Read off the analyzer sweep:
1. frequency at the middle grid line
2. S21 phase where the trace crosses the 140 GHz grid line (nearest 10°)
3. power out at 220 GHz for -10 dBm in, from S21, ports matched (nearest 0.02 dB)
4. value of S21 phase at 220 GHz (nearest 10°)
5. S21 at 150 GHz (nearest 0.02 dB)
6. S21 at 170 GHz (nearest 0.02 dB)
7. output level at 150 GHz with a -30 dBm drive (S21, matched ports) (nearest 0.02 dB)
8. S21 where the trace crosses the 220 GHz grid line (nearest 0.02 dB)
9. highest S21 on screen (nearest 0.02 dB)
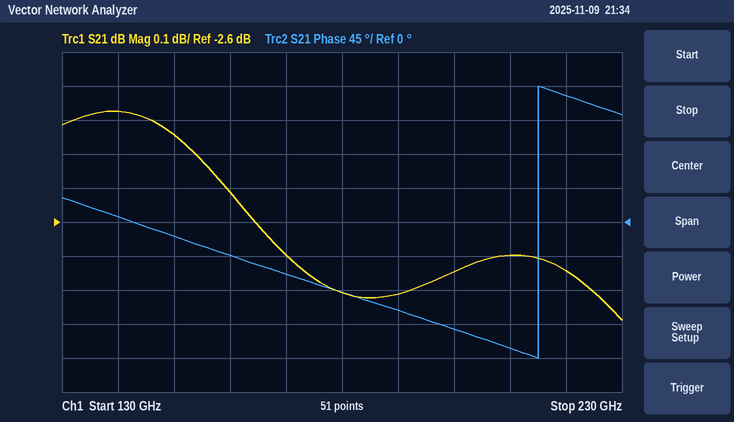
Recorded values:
180 GHz
10°
-12.74 dBm
170°
-2.34 dB
-2.70 dB
-32.34 dBm
-2.74 dB
-2.28 dB
